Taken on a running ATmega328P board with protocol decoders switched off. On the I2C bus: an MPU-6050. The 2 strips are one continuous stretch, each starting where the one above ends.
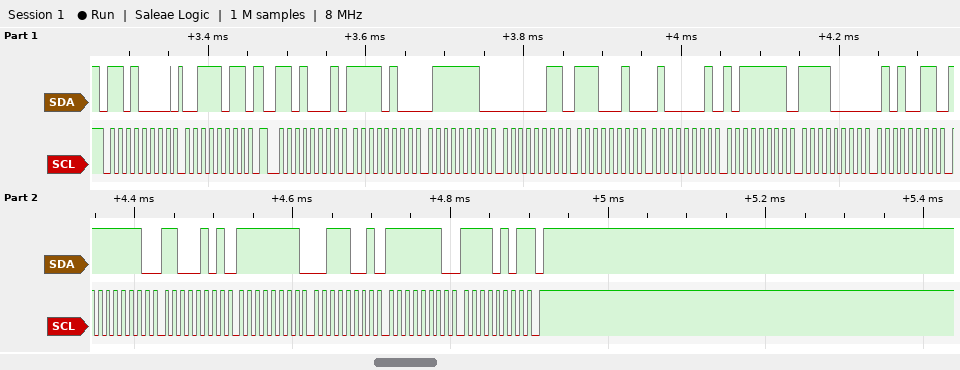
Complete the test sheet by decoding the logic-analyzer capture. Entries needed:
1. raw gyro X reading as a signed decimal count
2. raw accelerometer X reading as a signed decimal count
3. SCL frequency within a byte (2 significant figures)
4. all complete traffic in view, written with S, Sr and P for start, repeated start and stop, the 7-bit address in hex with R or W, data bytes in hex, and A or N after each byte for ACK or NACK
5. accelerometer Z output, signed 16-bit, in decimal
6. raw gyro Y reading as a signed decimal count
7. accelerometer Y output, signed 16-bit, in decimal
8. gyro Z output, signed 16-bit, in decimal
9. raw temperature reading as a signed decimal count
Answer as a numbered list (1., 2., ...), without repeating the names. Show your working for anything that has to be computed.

1. 0xFEC5 = -315
2. 0xF47E = -2946
3. 100 kHz
4. S 68W A 3B A Sr 68R A F4 A 7E A 03 A E2 A 41 A BF A F0 A 53 A FE A C5 A FF A 39 A FE A F5 N P
5. 0x41BF = 16831
6. 0xFF39 = -199
7. 0x03E2 = 994
8. 0xFEF5 = -267
9. 0xF053 = -4013
